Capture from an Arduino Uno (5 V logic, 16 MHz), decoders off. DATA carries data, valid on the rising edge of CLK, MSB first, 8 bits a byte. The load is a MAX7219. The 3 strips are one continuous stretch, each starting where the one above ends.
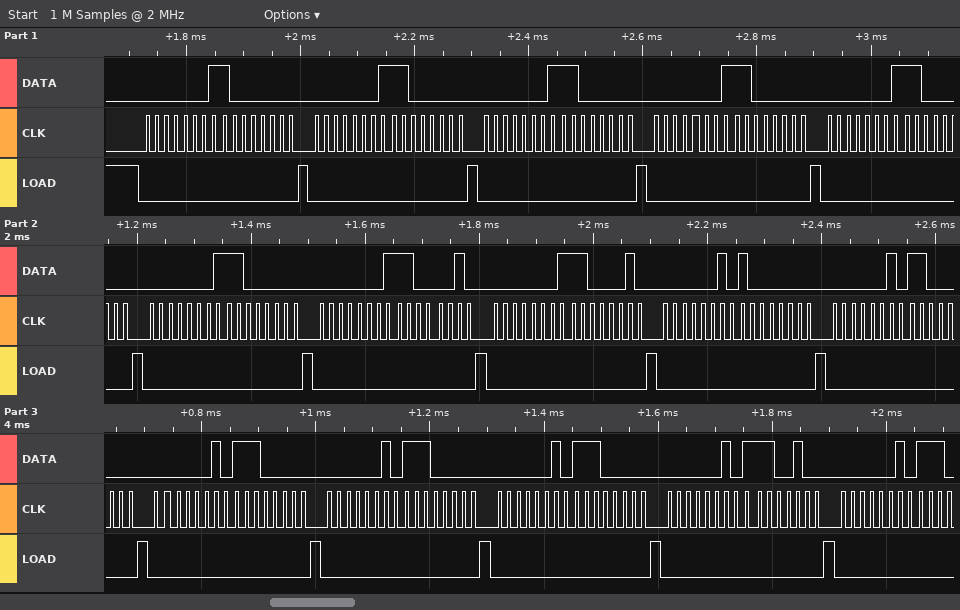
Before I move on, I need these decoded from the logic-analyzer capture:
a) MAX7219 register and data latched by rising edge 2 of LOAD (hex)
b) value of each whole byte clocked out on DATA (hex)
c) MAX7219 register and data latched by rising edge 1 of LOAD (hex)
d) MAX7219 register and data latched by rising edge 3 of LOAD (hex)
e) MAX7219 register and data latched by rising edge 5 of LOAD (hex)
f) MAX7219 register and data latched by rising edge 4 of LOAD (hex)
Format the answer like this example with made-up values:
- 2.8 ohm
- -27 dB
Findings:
- register 0x1, data 0xC0
- 01 80 01 C0 01 C0 01 C0 01 C0 01 C0 01 C2 01 C2 02 80 02 C0 02 E0 02 E0 02 E0 02 E4 02
- register 0x1, data 0x80
- register 0x1, data 0xC0
- register 0x1, data 0xC0
- register 0x1, data 0xC0
